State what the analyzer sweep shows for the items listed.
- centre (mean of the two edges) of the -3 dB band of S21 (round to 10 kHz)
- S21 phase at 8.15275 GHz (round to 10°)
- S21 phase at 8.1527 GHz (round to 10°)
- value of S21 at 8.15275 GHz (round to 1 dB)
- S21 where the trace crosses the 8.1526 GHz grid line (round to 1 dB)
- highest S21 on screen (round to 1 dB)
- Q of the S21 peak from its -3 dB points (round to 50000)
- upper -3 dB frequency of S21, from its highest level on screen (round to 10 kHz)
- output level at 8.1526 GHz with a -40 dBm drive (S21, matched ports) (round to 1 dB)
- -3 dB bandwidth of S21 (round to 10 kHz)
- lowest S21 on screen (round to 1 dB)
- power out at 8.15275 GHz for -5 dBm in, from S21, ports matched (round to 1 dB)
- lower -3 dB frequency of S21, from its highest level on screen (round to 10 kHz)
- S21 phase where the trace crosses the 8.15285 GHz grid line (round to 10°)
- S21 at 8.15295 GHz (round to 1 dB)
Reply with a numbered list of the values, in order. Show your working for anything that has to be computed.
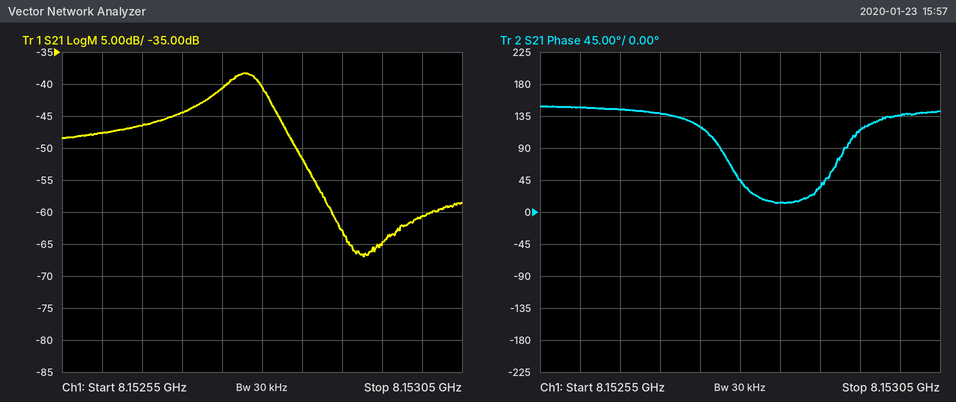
1. 8.15277 GHz
2. 120°
3. 140°
4. -41 dB
5. -48 dB
6. -38 dB
7. 8.15277 GHz / 60 kHz ≈ 135880, so 150000 to the nearest 50000
8. 8.15280 GHz
9. -40 dBm + (-48 dB) = -88 dBm
10. 8.15280 GHz − 8.15274 GHz = 60 kHz
11. -67 dB
12. -5 dBm + (-41 dB) = -46 dBm
13. 8.15274 GHz
14. 10°
15. -65 dB
